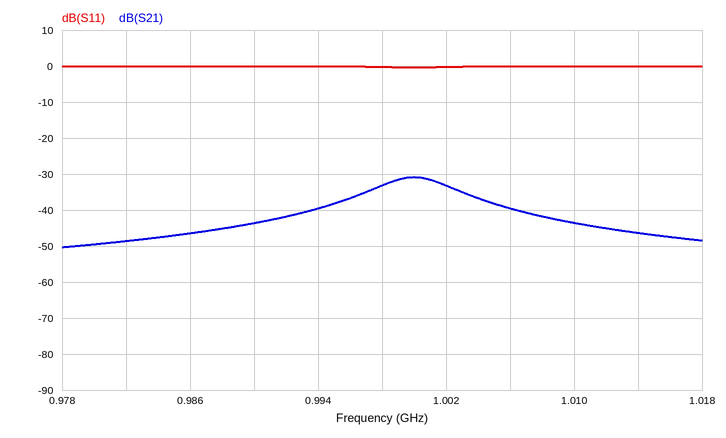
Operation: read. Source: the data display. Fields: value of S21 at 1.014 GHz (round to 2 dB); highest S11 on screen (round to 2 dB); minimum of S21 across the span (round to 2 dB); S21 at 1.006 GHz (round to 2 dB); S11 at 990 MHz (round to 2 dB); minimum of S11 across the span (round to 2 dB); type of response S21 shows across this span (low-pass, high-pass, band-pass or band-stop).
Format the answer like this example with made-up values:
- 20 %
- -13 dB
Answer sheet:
- -46 dB
- 0 dB
- -50 dB
- -40 dB
- 0 dB
- 0 dB
- band-pass
